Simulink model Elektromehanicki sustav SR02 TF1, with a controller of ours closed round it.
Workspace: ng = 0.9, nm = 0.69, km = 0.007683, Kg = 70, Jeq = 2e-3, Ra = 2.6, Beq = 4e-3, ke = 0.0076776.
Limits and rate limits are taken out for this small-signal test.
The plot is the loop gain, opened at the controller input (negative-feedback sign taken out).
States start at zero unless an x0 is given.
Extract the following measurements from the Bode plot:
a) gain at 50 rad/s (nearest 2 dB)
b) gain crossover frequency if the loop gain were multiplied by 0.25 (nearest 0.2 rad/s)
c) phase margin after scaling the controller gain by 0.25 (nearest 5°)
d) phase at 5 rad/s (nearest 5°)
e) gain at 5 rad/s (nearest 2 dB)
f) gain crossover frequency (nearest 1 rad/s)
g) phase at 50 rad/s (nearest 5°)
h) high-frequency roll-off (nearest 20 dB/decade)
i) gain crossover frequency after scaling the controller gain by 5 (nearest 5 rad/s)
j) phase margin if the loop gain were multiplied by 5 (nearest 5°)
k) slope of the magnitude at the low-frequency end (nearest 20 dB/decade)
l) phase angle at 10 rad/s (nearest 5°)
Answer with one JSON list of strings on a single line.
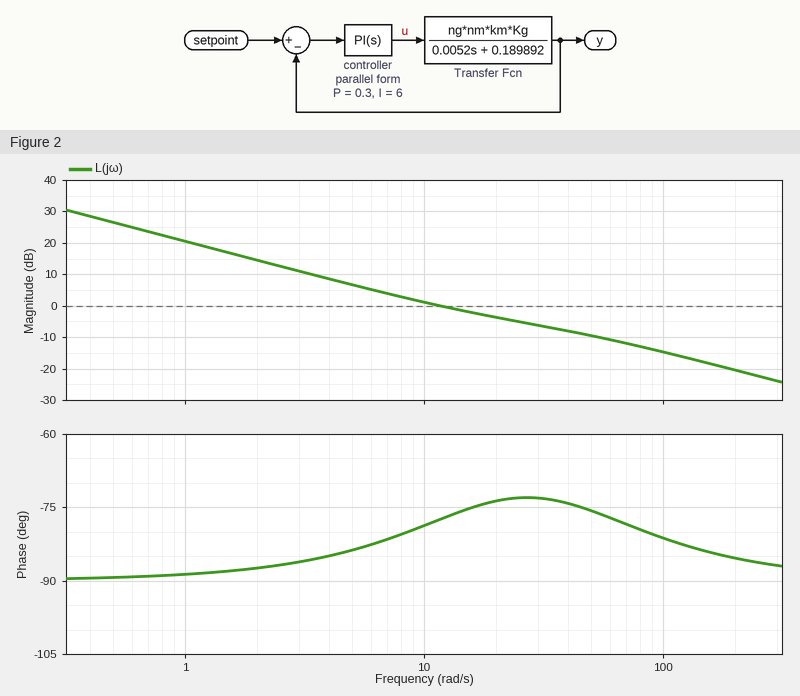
["-10 dB", "2.6 rad/s", "95°", "-85°", "6 dB", "12 rad/s", "-75°", "-20 dB/decade", "90 rad/s", "100°", "-20 dB/decade", "-80°"]
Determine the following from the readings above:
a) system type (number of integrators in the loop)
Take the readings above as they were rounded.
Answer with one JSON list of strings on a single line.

["1"]
